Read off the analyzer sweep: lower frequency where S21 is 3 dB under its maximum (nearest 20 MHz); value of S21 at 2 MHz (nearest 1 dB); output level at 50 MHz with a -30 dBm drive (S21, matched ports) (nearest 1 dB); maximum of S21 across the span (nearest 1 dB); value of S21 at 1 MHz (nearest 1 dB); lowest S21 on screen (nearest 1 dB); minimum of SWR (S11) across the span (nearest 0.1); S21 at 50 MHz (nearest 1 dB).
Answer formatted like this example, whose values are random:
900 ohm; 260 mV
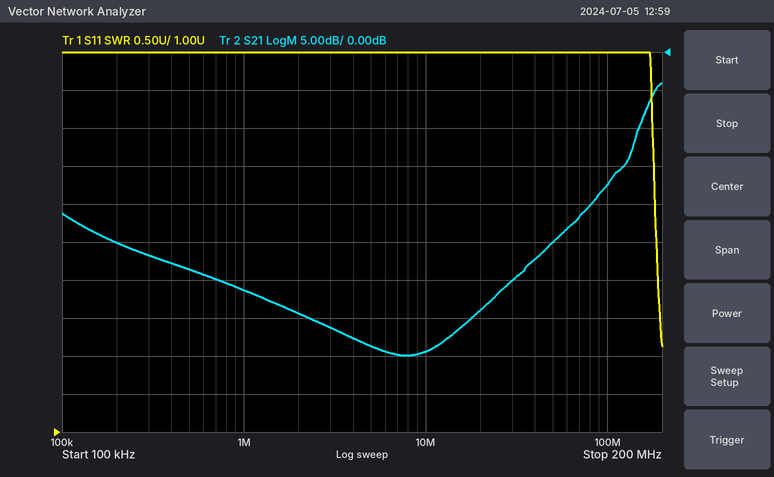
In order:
160 MHz; -34 dB; -55 dBm; -4 dB; -31 dB; -40 dB; 2.1; -25 dB
